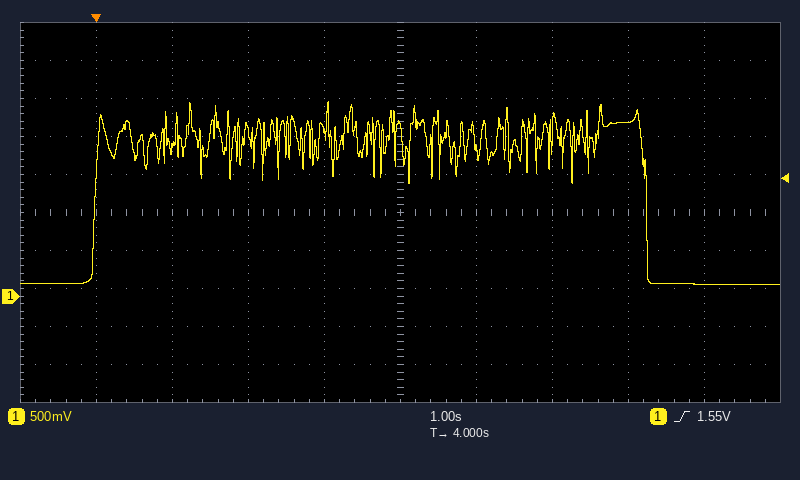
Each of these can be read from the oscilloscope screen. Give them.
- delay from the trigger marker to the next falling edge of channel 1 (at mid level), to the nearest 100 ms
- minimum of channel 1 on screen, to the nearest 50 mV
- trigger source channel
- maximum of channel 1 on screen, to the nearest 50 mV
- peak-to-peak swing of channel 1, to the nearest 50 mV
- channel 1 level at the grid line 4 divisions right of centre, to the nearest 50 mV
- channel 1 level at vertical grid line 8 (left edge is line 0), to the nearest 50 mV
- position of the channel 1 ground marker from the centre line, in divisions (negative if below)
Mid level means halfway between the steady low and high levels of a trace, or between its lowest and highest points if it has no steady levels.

7.2 s
150 mV
channel 1
2.55 V
2.40 V
150 mV
2.30 V
-2.2 div
